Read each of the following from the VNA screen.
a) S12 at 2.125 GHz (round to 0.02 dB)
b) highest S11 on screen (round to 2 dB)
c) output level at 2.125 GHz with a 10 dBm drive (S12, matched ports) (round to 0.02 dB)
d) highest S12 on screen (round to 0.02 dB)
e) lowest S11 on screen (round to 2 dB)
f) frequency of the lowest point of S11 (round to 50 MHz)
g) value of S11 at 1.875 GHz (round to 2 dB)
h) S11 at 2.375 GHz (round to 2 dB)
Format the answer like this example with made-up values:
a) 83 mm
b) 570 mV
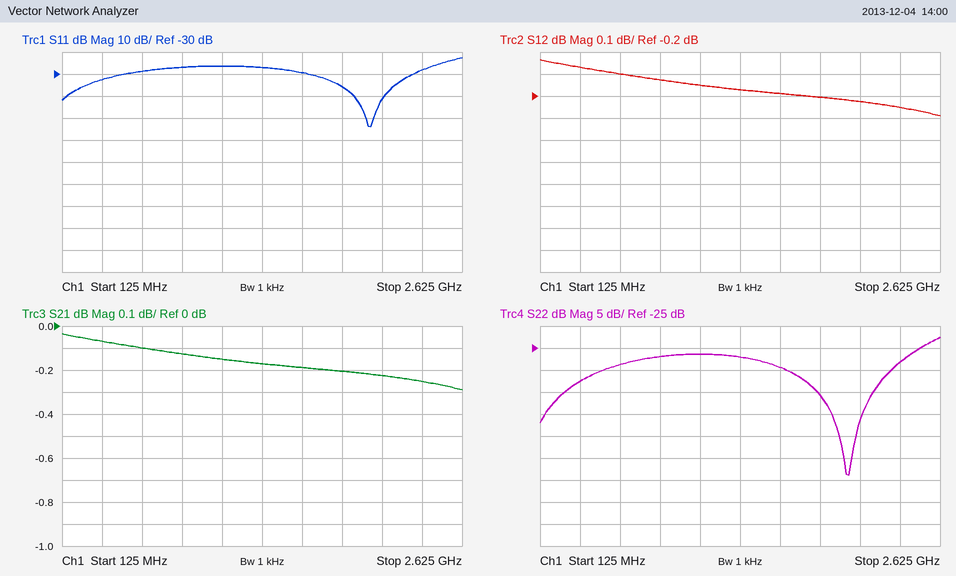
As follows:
a) -0.22 dB
b) -22 dB
c) 9.78 dBm
d) -0.04 dB
e) -54 dB
f) 2.05 GHz
g) -36 dB
h) -28 dB
